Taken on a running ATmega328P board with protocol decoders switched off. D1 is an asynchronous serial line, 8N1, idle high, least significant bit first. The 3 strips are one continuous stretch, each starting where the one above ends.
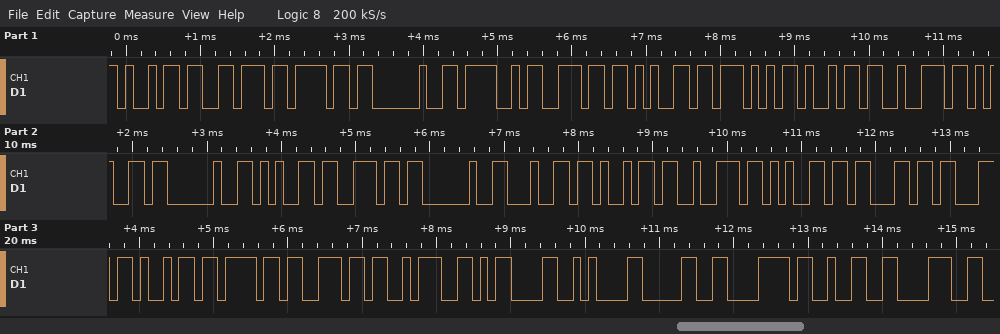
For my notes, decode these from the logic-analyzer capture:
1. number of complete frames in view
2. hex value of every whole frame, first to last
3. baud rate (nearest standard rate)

31
69 76 6F 20 4F 6E 65 57 69 72 65 20 65 6E 20 64 69 72 65 63 63 69 6F 6E 3A 0D 0A 30 78 32 38
9600 baud
